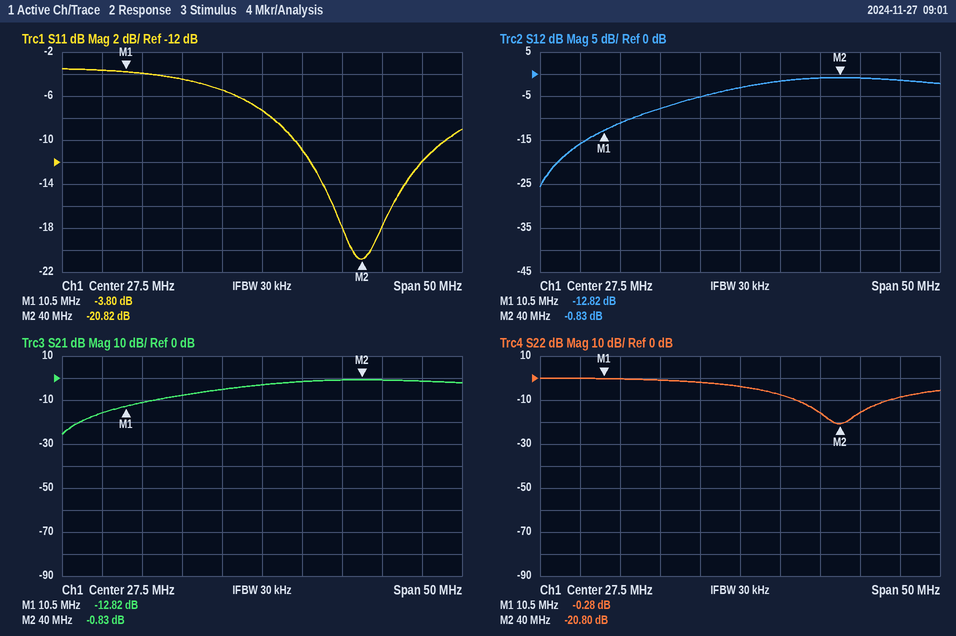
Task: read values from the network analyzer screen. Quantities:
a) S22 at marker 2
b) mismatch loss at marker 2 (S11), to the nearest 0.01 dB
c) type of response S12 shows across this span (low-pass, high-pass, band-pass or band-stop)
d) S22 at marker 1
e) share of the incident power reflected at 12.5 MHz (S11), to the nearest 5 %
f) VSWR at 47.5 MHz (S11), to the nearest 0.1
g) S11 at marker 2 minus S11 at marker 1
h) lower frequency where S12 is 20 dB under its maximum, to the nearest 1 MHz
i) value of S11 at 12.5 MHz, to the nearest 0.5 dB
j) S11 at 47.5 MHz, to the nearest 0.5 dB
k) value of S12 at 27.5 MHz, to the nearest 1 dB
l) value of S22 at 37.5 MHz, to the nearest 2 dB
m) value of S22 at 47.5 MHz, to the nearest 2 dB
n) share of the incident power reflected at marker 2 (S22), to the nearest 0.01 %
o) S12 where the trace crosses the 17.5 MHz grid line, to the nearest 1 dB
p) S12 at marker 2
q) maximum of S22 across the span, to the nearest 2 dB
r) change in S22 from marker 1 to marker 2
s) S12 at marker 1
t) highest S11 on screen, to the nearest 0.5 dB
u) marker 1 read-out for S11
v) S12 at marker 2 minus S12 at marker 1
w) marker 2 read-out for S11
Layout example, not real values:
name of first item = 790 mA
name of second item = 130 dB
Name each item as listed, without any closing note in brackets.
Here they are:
S22 at marker 2 = -20.80 dB
mismatch loss at marker 2 (S11), to the nearest 0.01 dB = 0.04 dB
type of response S12 shows across this span = high-pass
S22 at marker 1 = -0.28 dB
share of the incident power reflected at 12.5 MHz (S11), to the nearest 5 % = 40 %
VSWR at 47.5 MHz (S11), to the nearest 0.1 = 1.7
S11 at marker 2 minus S11 at marker 1 = -17.02 dB
lower frequency where S12 is 20 dB under its maximum, to the nearest 1 MHz = 4 MHz
value of S11 at 12.5 MHz, to the nearest 0.5 dB = -4.0 dB
S11 at 47.5 MHz, to the nearest 0.5 dB = -12.0 dB
value of S12 at 27.5 MHz, to the nearest 1 dB = -3 dB
value of S22 at 37.5 MHz, to the nearest 2 dB = -16 dB
value of S22 at 47.5 MHz, to the nearest 2 dB = -8 dB
share of the incident power reflected at marker 2 (S22), to the nearest 0.01 % = 0.83 %
S12 where the trace crosses the 17.5 MHz grid line, to the nearest 1 dB = -8 dB
S12 at marker 2 = -0.83 dB
maximum of S22 across the span, to the nearest 2 dB = 0 dB
change in S22 from marker 1 to marker 2 = -20.52 dB
S12 at marker 1 = -12.82 dB
highest S11 on screen, to the nearest 0.5 dB = -3.5 dB
marker 1 read-out for S11 = -3.80 dB
S12 at marker 2 minus S12 at marker 1 = 11.99 dB
marker 2 read-out for S11 = -20.82 dB
